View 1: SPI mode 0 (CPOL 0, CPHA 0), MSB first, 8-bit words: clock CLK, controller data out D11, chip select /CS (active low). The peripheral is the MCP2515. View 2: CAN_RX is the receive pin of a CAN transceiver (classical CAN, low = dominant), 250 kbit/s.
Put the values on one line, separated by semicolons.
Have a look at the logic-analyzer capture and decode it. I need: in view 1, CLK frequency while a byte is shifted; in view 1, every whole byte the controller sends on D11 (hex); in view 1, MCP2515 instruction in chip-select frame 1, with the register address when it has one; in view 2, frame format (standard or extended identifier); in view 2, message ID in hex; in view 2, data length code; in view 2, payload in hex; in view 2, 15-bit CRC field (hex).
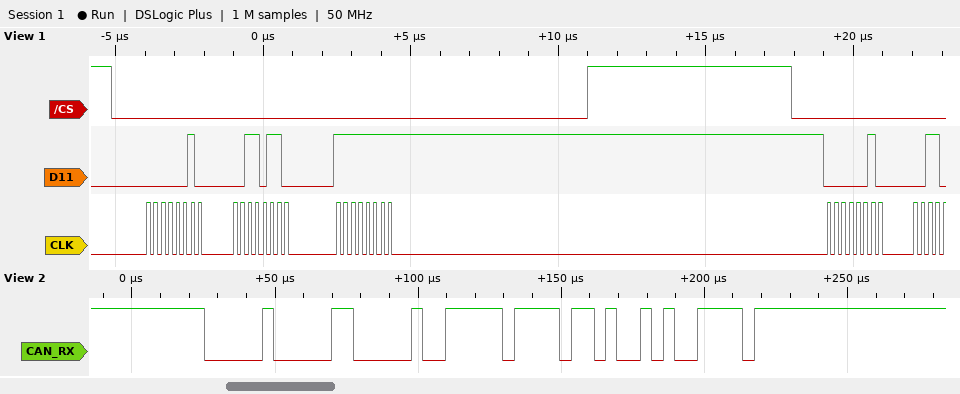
4 MHz; 02 36 FF 02; WRITE 0x36; standard; 0x002; 1; FF; 0x34A7
